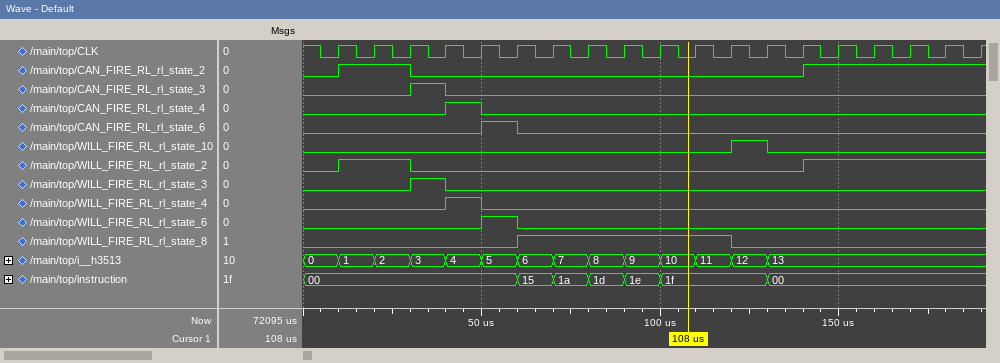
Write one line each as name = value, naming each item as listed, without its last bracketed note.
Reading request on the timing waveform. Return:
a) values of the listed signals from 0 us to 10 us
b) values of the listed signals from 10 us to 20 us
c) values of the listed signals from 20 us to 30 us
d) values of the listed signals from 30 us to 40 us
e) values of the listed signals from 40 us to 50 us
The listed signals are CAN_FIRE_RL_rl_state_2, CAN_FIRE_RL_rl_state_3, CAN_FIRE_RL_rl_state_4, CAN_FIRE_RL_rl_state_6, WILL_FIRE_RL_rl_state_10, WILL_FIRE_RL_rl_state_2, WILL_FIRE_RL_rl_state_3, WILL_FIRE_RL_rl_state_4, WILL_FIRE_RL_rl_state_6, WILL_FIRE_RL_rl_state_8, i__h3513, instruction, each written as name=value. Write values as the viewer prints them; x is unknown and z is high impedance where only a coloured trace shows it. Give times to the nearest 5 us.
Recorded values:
values of the listed signals from 0 us to 10 us = CAN_FIRE_RL_rl_state_2=0, CAN_FIRE_RL_rl_state_3=0, CAN_FIRE_RL_rl_state_4=0, CAN_FIRE_RL_rl_state_6=0, WILL_FIRE_RL_rl_state_10=0, WILL_FIRE_RL_rl_state_2=0, WILL_FIRE_RL_rl_state_3=0, WILL_FIRE_RL_rl_state_4=0, WILL_FIRE_RL_rl_state_6=0, WILL_FIRE_RL_rl_state_8=0, i__h3513=0, instruction=00
values of the listed signals from 10 us to 20 us = CAN_FIRE_RL_rl_state_2=1, CAN_FIRE_RL_rl_state_3=0, CAN_FIRE_RL_rl_state_4=0, CAN_FIRE_RL_rl_state_6=0, WILL_FIRE_RL_rl_state_10=0, WILL_FIRE_RL_rl_state_2=1, WILL_FIRE_RL_rl_state_3=0, WILL_FIRE_RL_rl_state_4=0, WILL_FIRE_RL_rl_state_6=0, WILL_FIRE_RL_rl_state_8=0, i__h3513=1, instruction=00
values of the listed signals from 20 us to 30 us = CAN_FIRE_RL_rl_state_2=1, CAN_FIRE_RL_rl_state_3=0, CAN_FIRE_RL_rl_state_4=0, CAN_FIRE_RL_rl_state_6=0, WILL_FIRE_RL_rl_state_10=0, WILL_FIRE_RL_rl_state_2=1, WILL_FIRE_RL_rl_state_3=0, WILL_FIRE_RL_rl_state_4=0, WILL_FIRE_RL_rl_state_6=0, WILL_FIRE_RL_rl_state_8=0, i__h3513=2, instruction=00
values of the listed signals from 30 us to 40 us = CAN_FIRE_RL_rl_state_2=0, CAN_FIRE_RL_rl_state_3=1, CAN_FIRE_RL_rl_state_4=0, CAN_FIRE_RL_rl_state_6=0, WILL_FIRE_RL_rl_state_10=0, WILL_FIRE_RL_rl_state_2=0, WILL_FIRE_RL_rl_state_3=1, WILL_FIRE_RL_rl_state_4=0, WILL_FIRE_RL_rl_state_6=0, WILL_FIRE_RL_rl_state_8=0, i__h3513=3, instruction=00
values of the listed signals from 40 us to 50 us = CAN_FIRE_RL_rl_state_2=0, CAN_FIRE_RL_rl_state_3=0, CAN_FIRE_RL_rl_state_4=1, CAN_FIRE_RL_rl_state_6=0, WILL_FIRE_RL_rl_state_10=0, WILL_FIRE_RL_rl_state_2=0, WILL_FIRE_RL_rl_state_3=0, WILL_FIRE_RL_rl_state_4=1, WILL_FIRE_RL_rl_state_6=0, WILL_FIRE_RL_rl_state_8=0, i__h3513=4, instruction=00
